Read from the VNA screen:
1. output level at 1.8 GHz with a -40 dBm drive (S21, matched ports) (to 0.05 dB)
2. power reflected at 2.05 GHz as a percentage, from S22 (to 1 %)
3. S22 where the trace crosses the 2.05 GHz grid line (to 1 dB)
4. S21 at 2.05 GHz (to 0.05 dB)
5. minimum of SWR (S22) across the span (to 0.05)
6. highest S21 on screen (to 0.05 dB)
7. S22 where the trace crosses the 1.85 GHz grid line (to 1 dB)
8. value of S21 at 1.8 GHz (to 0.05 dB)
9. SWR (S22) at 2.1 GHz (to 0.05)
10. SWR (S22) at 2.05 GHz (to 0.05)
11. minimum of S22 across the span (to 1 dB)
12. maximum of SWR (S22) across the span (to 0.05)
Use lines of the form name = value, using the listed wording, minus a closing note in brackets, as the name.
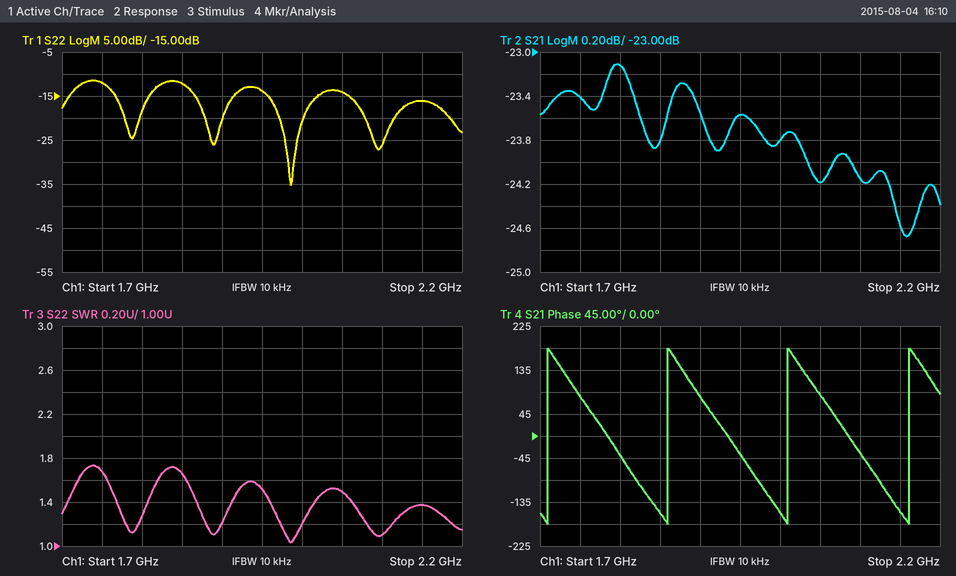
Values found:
output level at 1.8 GHz with a -40 dBm drive (S21, matched ports) = -63.10 dBm
power reflected at 2.05 GHz as a percentage, from S22 = 4 %
S22 where the trace crosses the 2.05 GHz grid line = -14 dB
S21 at 2.05 GHz = -24.20 dB
minimum of SWR (S22) across the span = 1.05
highest S21 on screen = -23.10 dB
S22 where the trace crosses the 1.85 GHz grid line = -12 dB
value of S21 at 1.8 GHz = -23.10 dB
SWR (S22) at 2.1 GHz = 1.10
SWR (S22) at 2.05 GHz = 1.50
minimum of S22 across the span = -35 dB
maximum of SWR (S22) across the span = 1.75
